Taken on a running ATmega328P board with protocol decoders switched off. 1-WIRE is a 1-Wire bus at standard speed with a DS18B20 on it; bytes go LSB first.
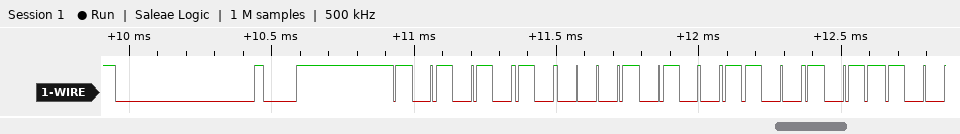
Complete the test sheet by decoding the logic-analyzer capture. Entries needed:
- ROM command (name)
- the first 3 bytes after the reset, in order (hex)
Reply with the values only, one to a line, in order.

Match ROM
55 28 D3
